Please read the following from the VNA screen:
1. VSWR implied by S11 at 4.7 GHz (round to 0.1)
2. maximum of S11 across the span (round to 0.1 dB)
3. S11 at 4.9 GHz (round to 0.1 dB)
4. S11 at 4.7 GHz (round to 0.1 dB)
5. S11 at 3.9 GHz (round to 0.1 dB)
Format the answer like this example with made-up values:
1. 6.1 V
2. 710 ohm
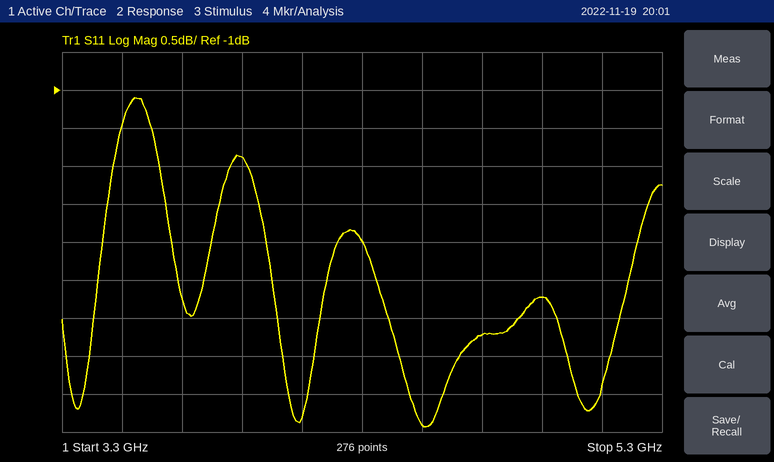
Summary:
1. 4.2
2. -1.1 dB
3. -3.7 dB
4. -4.2 dB
5. -1.9 dB
